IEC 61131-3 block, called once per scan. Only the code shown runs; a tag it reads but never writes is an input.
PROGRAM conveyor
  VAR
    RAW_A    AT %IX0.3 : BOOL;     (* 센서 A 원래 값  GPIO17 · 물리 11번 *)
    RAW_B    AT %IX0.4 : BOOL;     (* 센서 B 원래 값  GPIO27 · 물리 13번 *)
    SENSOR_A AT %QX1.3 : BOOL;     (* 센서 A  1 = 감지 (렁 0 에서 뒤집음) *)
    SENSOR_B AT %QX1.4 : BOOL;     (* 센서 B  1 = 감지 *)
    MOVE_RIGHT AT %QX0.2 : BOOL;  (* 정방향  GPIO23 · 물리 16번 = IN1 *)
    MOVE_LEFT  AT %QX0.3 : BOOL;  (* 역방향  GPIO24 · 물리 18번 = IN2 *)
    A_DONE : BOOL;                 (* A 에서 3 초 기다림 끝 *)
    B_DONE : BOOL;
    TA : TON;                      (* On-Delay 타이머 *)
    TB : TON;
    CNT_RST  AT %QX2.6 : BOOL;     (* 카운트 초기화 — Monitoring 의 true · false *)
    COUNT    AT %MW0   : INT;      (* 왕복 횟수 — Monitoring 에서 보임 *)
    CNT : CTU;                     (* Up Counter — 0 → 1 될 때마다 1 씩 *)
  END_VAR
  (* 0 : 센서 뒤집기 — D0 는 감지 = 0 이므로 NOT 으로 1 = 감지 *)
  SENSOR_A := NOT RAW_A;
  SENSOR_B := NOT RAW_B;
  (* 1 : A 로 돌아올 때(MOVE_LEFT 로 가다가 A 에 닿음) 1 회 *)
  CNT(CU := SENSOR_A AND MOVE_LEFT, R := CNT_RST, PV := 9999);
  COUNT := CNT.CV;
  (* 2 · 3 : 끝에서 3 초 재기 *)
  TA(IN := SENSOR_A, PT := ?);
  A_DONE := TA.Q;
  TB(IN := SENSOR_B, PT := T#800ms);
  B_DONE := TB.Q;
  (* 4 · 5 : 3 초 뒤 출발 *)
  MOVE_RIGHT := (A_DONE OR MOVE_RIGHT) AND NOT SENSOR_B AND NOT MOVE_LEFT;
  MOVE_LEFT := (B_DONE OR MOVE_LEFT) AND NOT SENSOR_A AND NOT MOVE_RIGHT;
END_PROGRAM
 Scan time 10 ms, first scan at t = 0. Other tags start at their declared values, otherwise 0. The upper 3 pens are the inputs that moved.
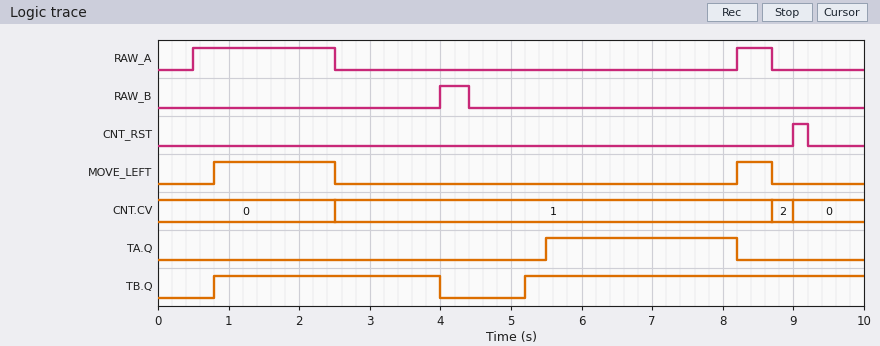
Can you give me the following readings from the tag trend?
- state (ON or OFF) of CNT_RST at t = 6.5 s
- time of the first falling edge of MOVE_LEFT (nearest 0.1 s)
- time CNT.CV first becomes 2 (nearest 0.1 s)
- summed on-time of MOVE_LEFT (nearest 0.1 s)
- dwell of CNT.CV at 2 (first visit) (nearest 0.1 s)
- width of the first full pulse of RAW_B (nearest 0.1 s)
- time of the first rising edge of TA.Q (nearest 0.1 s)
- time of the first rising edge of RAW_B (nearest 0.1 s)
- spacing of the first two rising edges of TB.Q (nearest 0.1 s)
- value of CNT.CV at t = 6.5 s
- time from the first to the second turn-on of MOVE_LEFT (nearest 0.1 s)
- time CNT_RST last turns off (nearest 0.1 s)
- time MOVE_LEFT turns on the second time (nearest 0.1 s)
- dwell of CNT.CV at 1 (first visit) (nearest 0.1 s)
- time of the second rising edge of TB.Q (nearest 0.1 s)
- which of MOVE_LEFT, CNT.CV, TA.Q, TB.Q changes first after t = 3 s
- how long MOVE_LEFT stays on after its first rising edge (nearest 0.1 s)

OFF
2.5 s
8.7 s
2.2 s
0.3 s
0.4 s
5.5 s
4.0 s
4.4 s
1
7.4 s
9.2 s
8.2 s
6.2 s
5.2 s
TB.Q
1.7 s
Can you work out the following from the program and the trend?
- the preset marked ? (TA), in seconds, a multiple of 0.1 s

3.0 s
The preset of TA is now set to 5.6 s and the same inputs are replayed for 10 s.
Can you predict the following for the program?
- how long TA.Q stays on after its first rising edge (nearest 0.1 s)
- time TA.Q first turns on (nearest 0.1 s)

0.1 s
8.1 s
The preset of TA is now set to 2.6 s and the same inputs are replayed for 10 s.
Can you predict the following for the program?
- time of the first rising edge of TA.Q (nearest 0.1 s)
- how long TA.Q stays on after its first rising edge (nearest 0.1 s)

5.1 s
3.1 s
